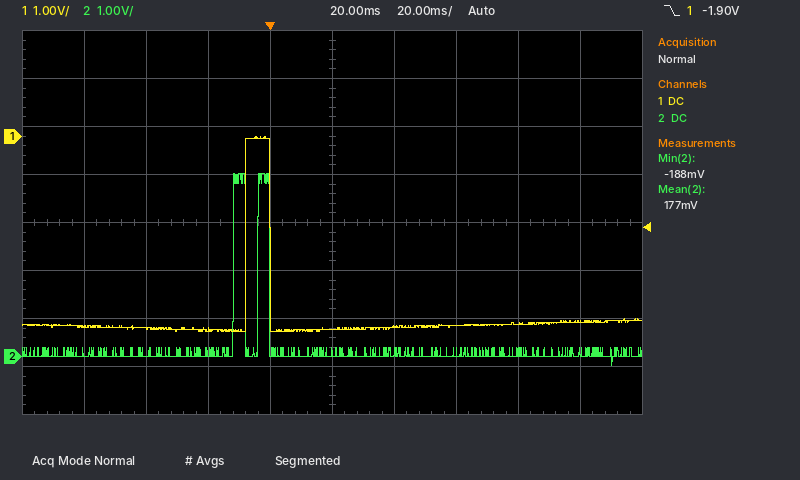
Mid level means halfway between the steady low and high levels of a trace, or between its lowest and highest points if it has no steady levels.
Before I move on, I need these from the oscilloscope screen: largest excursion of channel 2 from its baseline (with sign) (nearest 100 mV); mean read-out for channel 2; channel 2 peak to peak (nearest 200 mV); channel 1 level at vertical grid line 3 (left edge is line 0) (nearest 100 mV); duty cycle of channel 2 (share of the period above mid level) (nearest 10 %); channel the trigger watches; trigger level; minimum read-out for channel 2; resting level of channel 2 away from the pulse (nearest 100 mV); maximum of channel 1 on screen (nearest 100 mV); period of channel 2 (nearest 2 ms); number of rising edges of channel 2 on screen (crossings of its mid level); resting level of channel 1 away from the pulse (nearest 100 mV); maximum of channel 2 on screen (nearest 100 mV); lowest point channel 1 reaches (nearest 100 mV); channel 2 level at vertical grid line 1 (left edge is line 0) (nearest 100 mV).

+3.8 V
177 mV
4.0 V
-4.0 V
50 %
channel 1
-1.90 V
-188 mV
0.0 V
0.0 V
8 ms
2
-4.0 V
3.8 V
-4.1 V
100 mV
